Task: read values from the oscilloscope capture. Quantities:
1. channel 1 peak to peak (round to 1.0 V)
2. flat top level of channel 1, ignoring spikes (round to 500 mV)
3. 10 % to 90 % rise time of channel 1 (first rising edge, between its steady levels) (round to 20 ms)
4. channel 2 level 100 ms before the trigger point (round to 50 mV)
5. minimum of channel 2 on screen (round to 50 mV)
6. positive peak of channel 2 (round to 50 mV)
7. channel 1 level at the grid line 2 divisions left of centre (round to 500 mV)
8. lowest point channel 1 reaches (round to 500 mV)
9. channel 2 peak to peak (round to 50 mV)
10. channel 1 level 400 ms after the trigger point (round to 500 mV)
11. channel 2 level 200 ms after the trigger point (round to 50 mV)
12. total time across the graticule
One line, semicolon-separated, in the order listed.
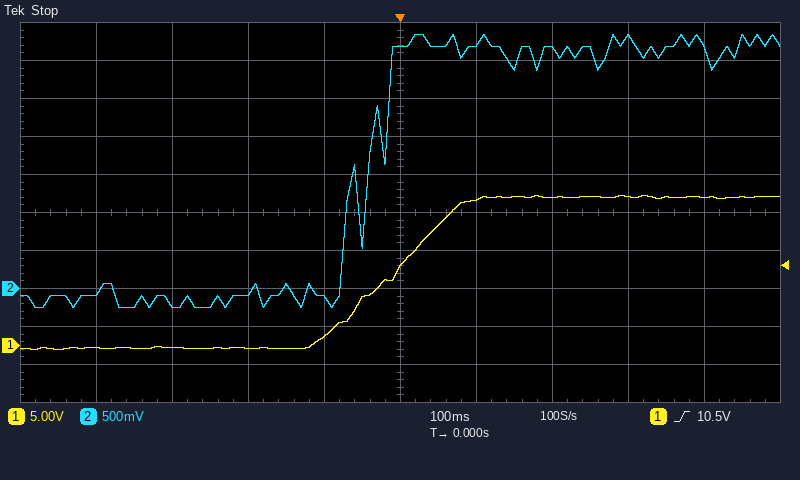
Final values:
20.0 V; 19.5 V; 160 ms; -150 mV; -250 mV; 3.35 V; -500 mV; -500 mV; 3.60 V; 19.5 V; 3.15 V; 1 s
